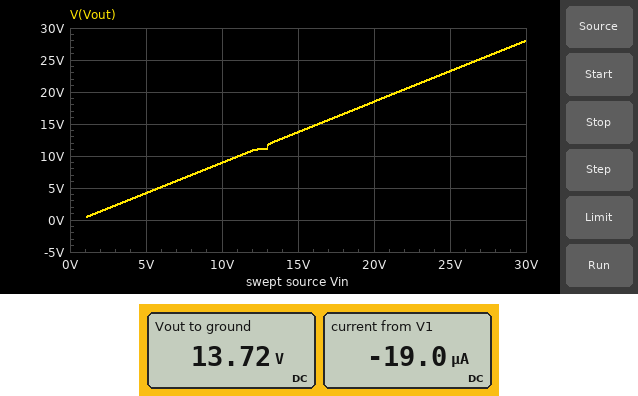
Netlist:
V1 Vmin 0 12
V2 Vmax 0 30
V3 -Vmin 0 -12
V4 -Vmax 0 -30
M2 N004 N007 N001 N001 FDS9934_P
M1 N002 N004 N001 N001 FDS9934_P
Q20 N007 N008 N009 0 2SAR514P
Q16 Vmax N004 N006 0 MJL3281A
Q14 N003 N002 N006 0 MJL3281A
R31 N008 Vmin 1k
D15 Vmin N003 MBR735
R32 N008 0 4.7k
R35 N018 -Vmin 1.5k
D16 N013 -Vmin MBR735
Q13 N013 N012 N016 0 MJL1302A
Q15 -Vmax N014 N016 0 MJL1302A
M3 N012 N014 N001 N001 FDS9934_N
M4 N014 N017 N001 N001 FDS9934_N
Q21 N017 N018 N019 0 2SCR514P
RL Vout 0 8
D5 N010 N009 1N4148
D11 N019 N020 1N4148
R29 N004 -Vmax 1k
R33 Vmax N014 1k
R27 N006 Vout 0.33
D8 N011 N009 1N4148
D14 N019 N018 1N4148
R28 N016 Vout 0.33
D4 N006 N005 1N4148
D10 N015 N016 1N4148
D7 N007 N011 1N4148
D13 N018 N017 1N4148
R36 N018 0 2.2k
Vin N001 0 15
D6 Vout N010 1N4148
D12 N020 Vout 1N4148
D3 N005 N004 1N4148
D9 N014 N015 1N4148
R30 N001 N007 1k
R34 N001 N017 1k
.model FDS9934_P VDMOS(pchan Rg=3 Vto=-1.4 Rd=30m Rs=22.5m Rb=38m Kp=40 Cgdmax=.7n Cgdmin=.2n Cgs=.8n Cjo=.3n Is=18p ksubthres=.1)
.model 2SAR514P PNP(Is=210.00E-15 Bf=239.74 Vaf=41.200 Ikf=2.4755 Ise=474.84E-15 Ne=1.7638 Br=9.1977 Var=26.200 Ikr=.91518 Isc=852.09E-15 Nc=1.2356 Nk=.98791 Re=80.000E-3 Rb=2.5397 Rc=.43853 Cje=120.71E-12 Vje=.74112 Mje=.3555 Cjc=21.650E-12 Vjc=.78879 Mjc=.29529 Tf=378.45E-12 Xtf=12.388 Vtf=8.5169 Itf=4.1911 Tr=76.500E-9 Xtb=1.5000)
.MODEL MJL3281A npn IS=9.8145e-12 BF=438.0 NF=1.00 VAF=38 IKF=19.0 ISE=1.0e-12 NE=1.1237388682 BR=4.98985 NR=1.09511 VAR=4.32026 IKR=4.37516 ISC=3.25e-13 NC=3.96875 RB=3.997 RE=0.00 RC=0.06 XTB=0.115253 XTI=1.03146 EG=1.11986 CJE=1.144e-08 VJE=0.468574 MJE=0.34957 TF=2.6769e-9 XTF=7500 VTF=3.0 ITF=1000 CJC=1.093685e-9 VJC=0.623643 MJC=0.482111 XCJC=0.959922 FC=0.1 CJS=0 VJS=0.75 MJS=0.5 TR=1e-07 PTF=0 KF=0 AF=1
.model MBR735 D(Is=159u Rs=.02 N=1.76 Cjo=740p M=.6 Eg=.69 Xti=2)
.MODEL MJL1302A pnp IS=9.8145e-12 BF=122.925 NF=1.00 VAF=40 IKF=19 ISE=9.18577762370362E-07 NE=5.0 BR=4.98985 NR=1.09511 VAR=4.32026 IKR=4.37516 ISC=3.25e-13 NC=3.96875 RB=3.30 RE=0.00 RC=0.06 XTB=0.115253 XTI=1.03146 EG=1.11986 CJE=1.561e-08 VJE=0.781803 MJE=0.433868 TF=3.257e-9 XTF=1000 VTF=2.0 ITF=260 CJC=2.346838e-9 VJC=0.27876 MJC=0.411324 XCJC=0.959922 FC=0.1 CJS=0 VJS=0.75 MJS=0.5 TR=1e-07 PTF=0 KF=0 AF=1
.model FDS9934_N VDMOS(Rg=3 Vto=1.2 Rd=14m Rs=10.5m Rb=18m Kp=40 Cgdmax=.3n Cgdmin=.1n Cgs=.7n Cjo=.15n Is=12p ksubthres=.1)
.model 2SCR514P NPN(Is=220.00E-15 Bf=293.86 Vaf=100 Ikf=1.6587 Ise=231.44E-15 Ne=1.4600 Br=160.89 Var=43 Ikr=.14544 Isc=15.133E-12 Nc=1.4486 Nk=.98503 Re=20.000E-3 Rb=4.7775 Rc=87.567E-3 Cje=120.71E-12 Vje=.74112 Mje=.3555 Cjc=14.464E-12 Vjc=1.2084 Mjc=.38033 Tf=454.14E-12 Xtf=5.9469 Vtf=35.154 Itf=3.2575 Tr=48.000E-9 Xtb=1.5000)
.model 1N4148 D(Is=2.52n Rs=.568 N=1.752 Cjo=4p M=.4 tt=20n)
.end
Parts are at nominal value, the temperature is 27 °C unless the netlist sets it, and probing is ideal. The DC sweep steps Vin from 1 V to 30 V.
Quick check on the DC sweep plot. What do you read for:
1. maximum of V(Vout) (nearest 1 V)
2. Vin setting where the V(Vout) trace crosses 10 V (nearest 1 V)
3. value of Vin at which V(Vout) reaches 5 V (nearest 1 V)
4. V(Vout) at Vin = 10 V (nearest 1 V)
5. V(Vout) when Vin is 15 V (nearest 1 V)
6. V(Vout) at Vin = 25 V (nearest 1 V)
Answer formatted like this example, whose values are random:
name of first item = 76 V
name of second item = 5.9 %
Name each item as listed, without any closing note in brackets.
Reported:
maximum of V(Vout) = 28 V
Vin setting where the V(Vout) trace crosses 10 V = 11 V
value of Vin at which V(Vout) reaches 5 V = 6 V
V(Vout) at Vin = 10 V = 9 V
V(Vout) when Vin is 15 V = 14 V
V(Vout) at Vin = 25 V = 23 V
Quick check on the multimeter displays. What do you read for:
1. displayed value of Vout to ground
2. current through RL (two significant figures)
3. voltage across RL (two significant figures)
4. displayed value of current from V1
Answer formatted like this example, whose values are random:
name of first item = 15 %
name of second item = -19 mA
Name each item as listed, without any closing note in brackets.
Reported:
displayed value of Vout to ground = 13.72 V
current through RL = 1.7 A
voltage across RL = 14 V
displayed value of current from V1 = -19.0 µA
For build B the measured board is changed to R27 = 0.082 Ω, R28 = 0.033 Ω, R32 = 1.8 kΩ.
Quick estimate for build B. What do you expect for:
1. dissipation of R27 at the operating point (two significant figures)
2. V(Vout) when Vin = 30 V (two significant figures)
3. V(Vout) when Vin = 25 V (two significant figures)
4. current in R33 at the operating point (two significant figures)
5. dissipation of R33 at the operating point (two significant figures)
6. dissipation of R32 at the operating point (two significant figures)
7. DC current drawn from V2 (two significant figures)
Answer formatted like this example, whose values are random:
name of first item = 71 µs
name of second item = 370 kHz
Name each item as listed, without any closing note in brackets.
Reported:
dissipation of R27 at the operating point = 250 mW
V(Vout) when Vin = 30 V = 29 V
V(Vout) when Vin = 25 V = 24 V
current in R33 at the operating point = 14 mA
dissipation of R33 at the operating point = 210 mW
dissipation of R32 at the operating point = 82 mW
DC current drawn from V2 = 1.8 A
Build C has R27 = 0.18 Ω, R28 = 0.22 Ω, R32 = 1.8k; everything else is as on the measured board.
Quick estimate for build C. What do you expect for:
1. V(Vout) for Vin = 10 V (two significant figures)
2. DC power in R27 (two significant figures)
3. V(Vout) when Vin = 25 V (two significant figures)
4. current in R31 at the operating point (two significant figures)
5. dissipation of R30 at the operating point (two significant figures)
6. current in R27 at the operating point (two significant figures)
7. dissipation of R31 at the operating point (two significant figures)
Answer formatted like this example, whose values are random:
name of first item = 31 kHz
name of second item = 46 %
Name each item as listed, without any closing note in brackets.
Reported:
V(Vout) for Vin = 10 V = 9.1 V
DC power in R27 = 540 mW
V(Vout) when Vin = 25 V = 24 V
current in R31 at the operating point = 33 µA
dissipation of R30 at the operating point = 5.5 mW
current in R27 at the operating point = 1.7 A
dissipation of R31 at the operating point = 1.1 µW
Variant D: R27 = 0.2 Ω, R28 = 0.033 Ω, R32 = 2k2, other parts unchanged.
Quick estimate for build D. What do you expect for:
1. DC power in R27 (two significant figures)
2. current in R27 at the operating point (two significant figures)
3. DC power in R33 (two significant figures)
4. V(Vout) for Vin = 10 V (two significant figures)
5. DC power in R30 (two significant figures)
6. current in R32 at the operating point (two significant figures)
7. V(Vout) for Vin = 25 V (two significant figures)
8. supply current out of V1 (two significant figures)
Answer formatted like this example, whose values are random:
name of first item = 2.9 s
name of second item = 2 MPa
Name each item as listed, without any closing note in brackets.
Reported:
DC power in R27 = 600 mW
current in R27 at the operating point = 1.7 A
DC power in R33 = 210 mW
V(Vout) for Vin = 10 V = 9.1 V
DC power in R30 = 5.5 mW
current in R32 at the operating point = 5.4 mA
V(Vout) for Vin = 25 V = 24 V
supply current out of V1 = 26 µA
